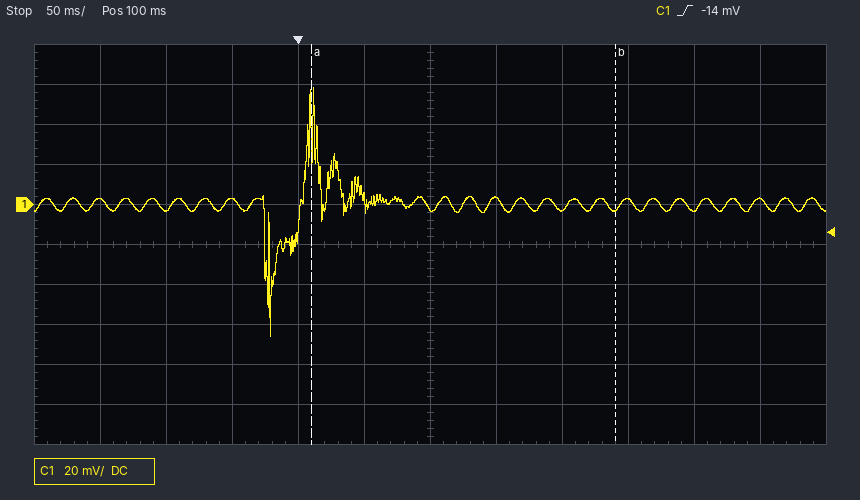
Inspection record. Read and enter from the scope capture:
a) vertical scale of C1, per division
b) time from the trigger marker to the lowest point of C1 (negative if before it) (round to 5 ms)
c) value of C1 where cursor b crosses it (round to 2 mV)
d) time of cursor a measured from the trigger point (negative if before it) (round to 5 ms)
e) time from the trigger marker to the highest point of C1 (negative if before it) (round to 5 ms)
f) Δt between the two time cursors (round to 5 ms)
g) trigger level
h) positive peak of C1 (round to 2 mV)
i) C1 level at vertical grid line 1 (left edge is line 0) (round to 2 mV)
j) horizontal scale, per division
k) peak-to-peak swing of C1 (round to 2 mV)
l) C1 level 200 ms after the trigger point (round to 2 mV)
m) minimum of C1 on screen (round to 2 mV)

20 mV
-20 ms
-2 mV
+10 ms
+10 ms
230 ms
-14 mV
58 mV
2 mV
50 ms
124 mV
-2 mV
-66 mV
